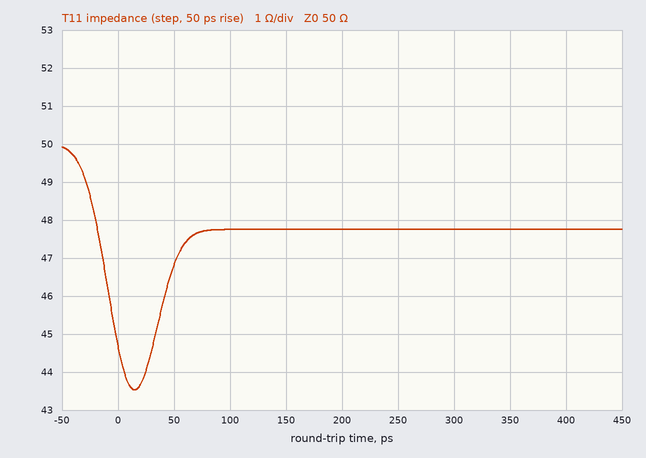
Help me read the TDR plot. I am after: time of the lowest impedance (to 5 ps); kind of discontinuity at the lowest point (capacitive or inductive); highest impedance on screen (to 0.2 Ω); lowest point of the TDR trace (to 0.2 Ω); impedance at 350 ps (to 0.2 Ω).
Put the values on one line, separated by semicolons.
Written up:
15 ps; capacitive; 50.0 Ω; 43.6 Ω; 47.8 Ω
